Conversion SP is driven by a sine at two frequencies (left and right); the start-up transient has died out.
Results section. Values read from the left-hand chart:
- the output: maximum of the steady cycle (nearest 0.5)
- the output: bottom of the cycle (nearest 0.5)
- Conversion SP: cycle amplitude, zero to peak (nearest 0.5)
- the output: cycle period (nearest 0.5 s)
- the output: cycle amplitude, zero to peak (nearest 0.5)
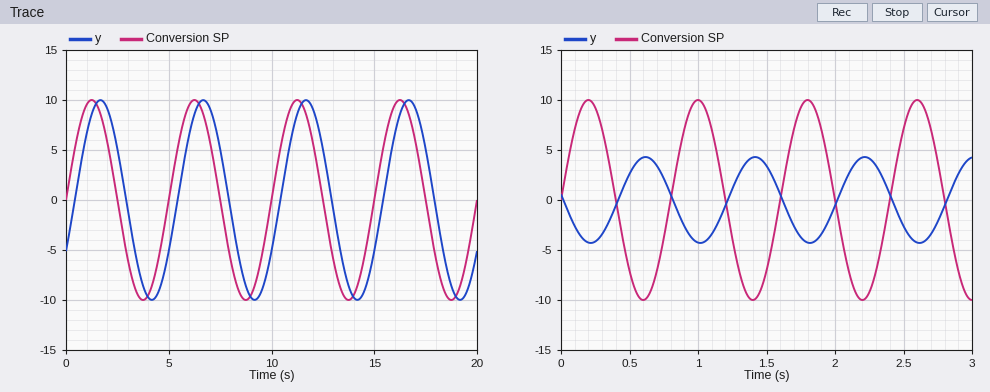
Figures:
10.0
-10.0
10.0
5.0 s
10.0
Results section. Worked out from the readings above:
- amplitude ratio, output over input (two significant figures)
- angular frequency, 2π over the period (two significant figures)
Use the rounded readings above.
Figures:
1.0
1.3 rad/s
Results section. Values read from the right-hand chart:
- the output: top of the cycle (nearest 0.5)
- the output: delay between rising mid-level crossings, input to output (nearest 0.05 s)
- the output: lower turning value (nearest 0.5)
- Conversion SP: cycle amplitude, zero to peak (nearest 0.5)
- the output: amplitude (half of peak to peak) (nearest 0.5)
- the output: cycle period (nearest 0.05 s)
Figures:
4.5
0.40 s
-4.5
10.0
4.5
0.80 s
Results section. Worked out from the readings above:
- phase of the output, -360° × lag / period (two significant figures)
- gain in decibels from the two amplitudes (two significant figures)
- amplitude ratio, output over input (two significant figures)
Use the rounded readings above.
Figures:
-180°
-6.9 dB
0.45
